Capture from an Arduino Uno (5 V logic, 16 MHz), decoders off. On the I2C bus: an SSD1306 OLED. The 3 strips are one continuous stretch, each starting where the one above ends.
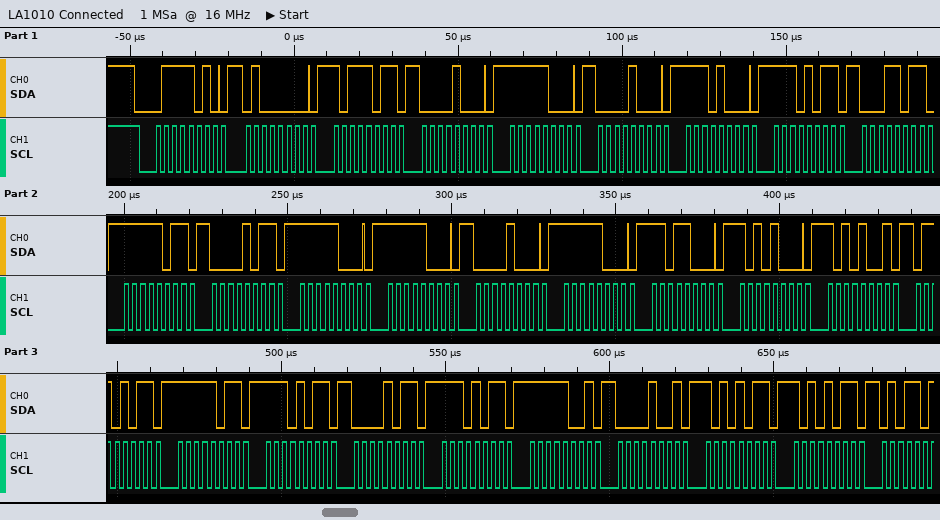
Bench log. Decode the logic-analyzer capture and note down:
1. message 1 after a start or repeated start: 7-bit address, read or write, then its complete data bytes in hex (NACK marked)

0x3D write: 40 BB 08 F8 08 E8 EB 1B FB 0B F8 F8 08 F8 D8 A8 A9 6B FB EB 0B EB F9 09 AB AB
